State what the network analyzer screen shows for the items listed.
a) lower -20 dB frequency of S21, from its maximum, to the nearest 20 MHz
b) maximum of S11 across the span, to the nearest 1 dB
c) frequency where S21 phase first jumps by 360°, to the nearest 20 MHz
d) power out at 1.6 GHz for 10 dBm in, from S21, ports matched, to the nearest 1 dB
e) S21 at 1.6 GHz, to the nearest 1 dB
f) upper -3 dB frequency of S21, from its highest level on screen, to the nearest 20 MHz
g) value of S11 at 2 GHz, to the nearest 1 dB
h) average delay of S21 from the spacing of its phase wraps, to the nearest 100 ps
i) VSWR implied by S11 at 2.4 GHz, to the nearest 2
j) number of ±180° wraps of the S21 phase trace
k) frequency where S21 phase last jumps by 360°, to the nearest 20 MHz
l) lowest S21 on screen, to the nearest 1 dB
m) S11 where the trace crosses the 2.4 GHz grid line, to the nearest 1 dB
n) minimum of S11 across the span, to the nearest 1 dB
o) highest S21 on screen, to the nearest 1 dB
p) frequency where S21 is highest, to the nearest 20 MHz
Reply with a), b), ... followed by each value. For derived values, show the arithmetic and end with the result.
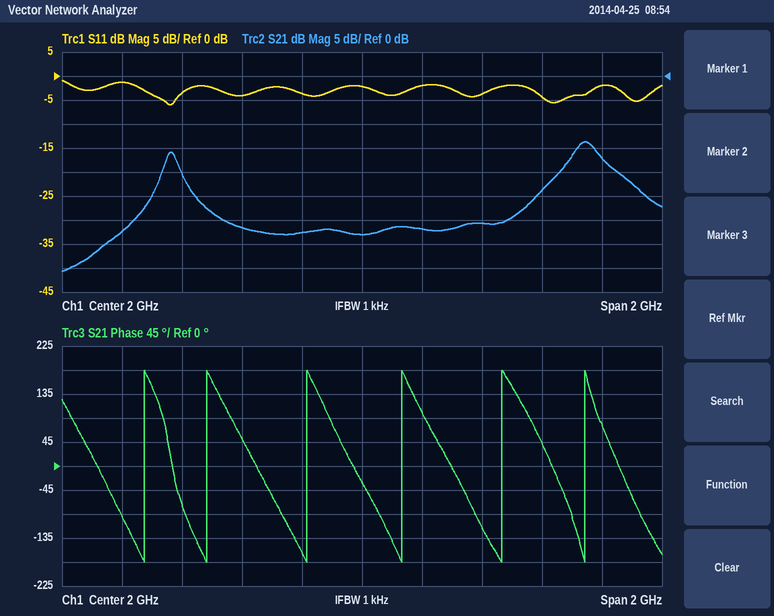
a) 1.18 GHz
b) -1 dB
c) 1.28 GHz
d) 10 dBm + (-32 dB) = -22 dBm
e) -32 dB
f) 2.80 GHz
g) -2 dB
h) 5 cycles / (2.74 GHz − 1.28 GHz) ≈ 3.4 ns
i) |Γ| = 10^(-4/20) = 0.6310; VSWR = (1 + 0.6310)/(1 − 0.6310) ≈ 4
j) 6
k) 2.74 GHz
l) -41 dB
m) -4 dB
n) -6 dB
o) -14 dB
p) 2.74 GHz
